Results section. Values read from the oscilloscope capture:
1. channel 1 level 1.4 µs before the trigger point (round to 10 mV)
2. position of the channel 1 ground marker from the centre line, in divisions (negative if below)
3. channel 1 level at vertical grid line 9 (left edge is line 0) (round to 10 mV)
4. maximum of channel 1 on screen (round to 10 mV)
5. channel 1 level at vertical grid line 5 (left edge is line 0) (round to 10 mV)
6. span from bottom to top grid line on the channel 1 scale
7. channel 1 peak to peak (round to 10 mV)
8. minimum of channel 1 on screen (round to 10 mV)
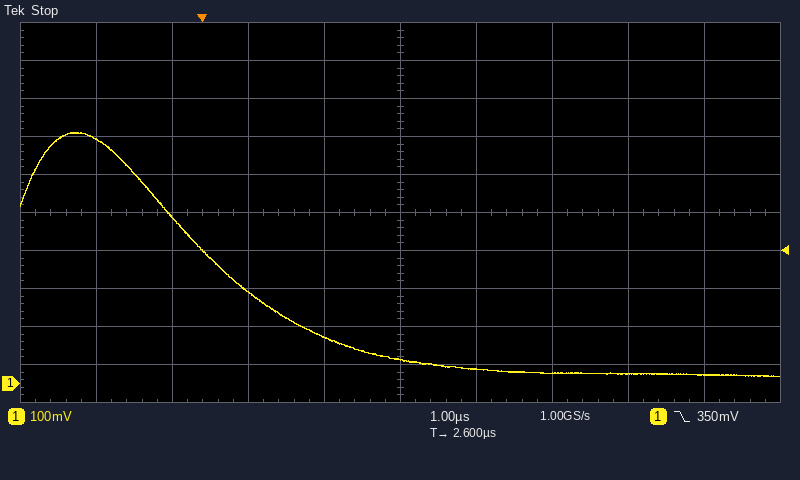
640 mV
-4.5 div
20 mV
660 mV
60 mV
1 V
640 mV
20 mV
